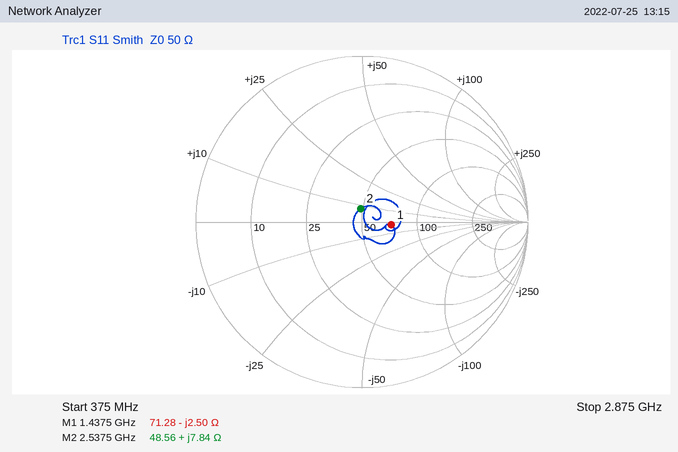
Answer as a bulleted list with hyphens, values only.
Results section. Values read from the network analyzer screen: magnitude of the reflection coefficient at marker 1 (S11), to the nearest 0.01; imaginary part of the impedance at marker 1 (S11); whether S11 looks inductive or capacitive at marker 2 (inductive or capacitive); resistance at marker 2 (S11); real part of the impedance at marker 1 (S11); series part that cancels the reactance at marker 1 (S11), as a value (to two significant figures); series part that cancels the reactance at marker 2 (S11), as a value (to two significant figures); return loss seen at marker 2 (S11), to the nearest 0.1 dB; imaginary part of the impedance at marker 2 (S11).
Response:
- 0.18
- -2.50 Ω
- inductive
- 48.56 Ω
- 71.28 Ω
- 280 pH
- 8.0 pF
- 21.9 dB
- +7.84 Ω
